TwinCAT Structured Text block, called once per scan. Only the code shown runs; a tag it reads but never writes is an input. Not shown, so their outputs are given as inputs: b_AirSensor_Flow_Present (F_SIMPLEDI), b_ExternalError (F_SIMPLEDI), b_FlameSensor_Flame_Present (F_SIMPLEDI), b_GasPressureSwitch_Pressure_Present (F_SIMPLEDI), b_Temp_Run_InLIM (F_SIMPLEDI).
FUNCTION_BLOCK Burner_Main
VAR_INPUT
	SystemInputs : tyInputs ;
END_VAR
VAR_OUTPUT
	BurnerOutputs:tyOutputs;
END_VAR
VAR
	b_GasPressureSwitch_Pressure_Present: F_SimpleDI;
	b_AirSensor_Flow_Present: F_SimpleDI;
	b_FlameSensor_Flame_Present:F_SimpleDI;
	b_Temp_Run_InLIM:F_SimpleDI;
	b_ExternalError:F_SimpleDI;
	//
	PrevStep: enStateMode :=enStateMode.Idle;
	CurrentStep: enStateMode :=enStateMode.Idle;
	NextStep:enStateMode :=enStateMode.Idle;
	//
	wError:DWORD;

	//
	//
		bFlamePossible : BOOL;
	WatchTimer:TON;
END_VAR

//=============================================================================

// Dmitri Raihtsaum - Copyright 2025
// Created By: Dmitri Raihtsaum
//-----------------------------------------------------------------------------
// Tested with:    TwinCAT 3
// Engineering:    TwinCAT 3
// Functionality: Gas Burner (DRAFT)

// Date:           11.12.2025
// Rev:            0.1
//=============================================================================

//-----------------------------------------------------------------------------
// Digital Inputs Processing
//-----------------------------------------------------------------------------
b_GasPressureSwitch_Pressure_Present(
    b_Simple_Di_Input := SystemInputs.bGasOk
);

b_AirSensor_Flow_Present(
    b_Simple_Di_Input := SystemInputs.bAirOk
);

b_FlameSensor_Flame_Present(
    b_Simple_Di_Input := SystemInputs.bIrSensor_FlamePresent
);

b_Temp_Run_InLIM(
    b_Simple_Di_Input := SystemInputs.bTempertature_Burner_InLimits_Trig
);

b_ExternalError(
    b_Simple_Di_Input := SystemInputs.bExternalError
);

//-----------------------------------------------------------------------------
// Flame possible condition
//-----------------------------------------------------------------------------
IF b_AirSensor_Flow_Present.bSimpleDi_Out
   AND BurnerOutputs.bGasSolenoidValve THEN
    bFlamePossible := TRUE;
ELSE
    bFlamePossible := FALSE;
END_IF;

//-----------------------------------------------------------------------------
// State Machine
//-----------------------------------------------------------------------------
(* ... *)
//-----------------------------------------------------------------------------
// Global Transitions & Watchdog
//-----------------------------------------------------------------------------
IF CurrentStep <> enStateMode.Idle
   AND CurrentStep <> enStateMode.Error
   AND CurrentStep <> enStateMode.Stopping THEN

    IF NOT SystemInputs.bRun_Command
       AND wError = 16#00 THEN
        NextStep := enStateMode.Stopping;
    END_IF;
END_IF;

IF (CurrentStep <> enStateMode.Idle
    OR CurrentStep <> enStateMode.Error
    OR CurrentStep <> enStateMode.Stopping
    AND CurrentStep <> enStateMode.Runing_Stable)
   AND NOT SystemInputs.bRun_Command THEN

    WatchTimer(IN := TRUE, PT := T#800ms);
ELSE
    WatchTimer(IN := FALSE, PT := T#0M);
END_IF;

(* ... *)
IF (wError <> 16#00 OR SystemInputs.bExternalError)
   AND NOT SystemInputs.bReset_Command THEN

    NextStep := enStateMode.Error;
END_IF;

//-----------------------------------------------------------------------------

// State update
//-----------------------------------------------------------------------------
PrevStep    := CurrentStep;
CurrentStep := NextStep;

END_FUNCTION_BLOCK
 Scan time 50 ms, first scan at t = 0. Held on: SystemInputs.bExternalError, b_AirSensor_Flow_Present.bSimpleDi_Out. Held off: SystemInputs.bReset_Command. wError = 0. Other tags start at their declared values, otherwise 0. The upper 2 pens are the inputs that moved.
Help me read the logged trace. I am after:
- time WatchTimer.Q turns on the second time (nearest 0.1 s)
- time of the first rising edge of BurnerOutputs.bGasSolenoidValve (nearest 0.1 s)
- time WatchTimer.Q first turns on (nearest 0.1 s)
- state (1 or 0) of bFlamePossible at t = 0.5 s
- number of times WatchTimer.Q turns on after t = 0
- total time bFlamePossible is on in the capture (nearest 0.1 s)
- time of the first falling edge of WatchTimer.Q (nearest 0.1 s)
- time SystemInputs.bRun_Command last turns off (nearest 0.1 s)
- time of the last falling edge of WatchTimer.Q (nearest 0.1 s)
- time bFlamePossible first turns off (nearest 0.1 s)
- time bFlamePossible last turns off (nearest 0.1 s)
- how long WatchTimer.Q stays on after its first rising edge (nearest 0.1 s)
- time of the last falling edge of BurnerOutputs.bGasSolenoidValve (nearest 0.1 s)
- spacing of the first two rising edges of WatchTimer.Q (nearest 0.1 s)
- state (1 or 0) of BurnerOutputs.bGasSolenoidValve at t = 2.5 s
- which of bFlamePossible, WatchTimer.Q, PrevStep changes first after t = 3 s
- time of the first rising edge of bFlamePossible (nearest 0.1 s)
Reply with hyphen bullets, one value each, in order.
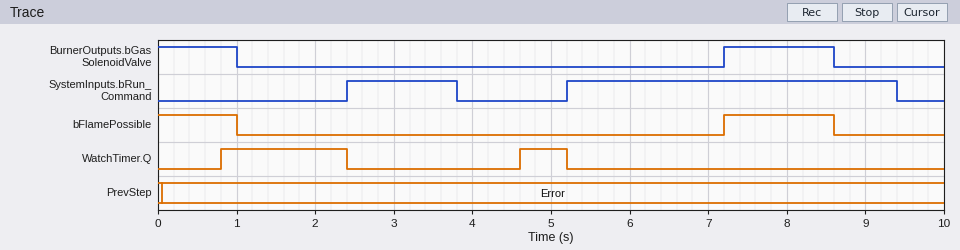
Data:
- 4.6 s
- 7.2 s
- 0.8 s
- 1
- 2
- 2.4 s
- 2.4 s
- 9.4 s
- 5.2 s
- 1.0 s
- 8.6 s
- 1.6 s
- 8.6 s
- 3.8 s
- 0
- WatchTimer.Q
- 7.2 s
